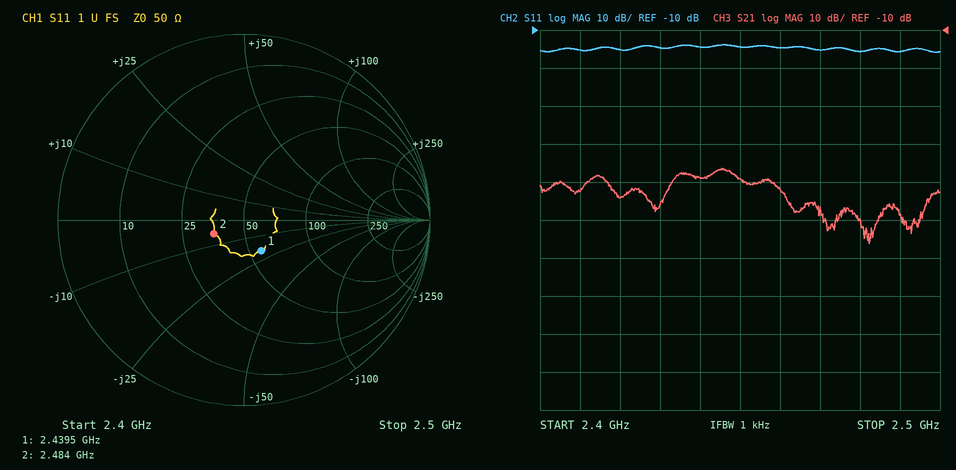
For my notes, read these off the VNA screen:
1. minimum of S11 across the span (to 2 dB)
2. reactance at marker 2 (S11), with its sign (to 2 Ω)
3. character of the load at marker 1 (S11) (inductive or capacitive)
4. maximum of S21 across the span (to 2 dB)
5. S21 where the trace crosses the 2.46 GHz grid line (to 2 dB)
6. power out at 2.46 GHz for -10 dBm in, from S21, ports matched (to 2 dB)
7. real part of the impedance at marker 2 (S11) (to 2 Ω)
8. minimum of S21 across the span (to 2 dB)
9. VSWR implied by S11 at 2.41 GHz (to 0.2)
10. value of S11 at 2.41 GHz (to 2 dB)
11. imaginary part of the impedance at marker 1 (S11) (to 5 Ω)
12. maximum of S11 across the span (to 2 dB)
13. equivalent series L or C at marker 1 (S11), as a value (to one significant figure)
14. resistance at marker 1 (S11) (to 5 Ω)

-16 dB
-6 Ω
capacitive
-46 dB
-52 dB
-62 dBm
36 Ω
-66 dB
1.4
-16 dB
-20 Ω
-14 dB
3 pF
55 Ω
